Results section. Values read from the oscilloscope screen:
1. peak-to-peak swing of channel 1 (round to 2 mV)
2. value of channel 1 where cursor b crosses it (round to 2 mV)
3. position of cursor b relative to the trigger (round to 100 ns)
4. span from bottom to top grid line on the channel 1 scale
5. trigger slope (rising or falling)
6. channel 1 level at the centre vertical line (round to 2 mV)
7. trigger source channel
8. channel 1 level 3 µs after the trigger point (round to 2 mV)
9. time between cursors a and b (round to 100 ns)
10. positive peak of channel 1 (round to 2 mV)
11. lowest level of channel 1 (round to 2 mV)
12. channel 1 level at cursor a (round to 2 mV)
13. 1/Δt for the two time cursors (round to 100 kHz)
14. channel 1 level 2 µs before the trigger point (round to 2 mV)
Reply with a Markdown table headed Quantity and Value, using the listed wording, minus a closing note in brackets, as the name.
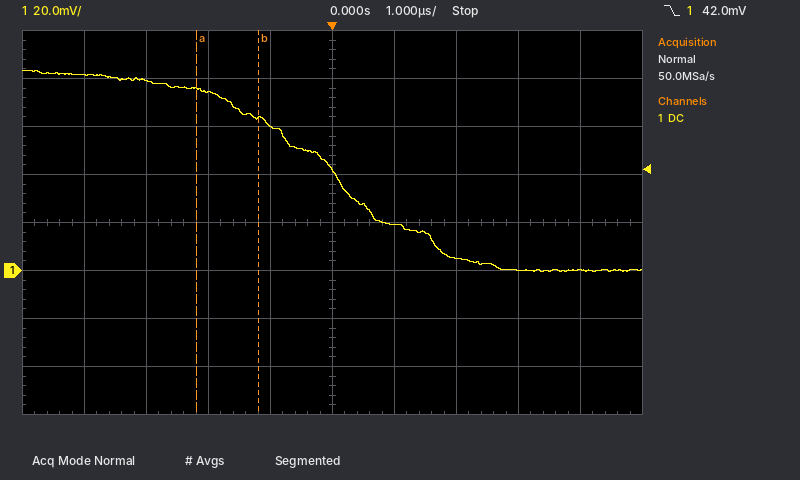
| Quantity | Value |
|---|---|
| peak-to-peak swing of channel 1 | 84 mV |
| value of channel 1 where cursor b crosses it | 64 mV |
| position of cursor b relative to the trigger | -1.2 µs |
| span from bottom to top grid line on the channel 1 scale | 160 mV |
| trigger slope | falling |
| channel 1 level at the centre vertical line | 42 mV |
| trigger source channel | channel 1 |
| channel 1 level 3 µs after the trigger point | 0 mV |
| time between cursors a and b | 1.0 µs |
| positive peak of channel 1 | 84 mV |
| lowest level of channel 1 | 0 mV |
| channel 1 level at cursor a | 76 mV |
| 1/Δt for the two time cursors | 1.0 MHz |
| channel 1 level 2 µs before the trigger point | 74 mV |
